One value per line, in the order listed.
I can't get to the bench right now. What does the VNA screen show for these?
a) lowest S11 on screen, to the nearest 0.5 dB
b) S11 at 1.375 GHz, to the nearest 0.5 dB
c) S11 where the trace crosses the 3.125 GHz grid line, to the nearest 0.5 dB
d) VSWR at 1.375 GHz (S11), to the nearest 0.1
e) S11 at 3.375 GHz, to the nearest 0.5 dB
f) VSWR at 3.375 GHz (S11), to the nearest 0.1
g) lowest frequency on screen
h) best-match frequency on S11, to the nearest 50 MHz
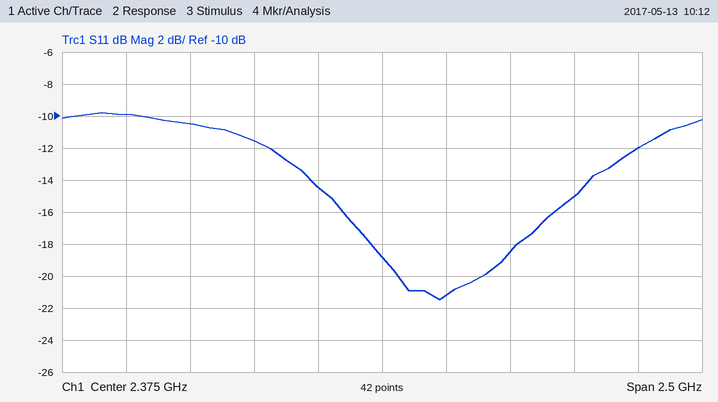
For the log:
-21.5 dB
-10.0 dB
-15.0 dB
1.9
-12.0 dB
1.7
1.125 GHz
2.60 GHz
